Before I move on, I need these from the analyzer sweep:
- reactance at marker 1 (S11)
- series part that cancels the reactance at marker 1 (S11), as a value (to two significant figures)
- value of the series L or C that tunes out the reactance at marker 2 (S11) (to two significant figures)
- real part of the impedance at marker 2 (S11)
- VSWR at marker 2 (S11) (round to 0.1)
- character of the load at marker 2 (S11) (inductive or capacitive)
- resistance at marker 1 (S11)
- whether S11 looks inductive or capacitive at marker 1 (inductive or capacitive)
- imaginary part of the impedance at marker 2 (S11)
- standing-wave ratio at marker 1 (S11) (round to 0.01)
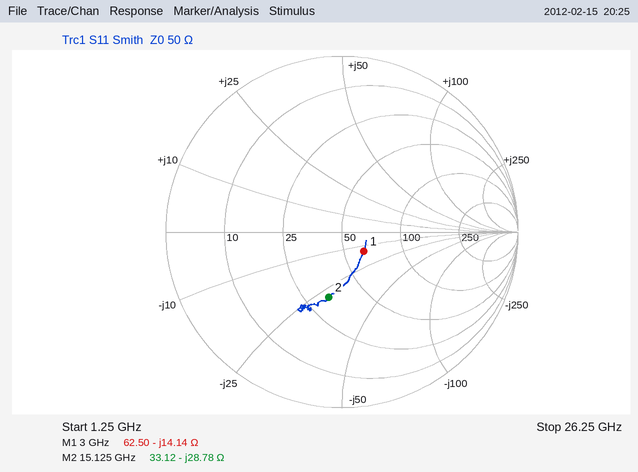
-14.14 Ω
750 pH
300 pH
33.12 Ω
2.2
capacitive
62.50 Ω
capacitive
-28.78 Ω
1.40
